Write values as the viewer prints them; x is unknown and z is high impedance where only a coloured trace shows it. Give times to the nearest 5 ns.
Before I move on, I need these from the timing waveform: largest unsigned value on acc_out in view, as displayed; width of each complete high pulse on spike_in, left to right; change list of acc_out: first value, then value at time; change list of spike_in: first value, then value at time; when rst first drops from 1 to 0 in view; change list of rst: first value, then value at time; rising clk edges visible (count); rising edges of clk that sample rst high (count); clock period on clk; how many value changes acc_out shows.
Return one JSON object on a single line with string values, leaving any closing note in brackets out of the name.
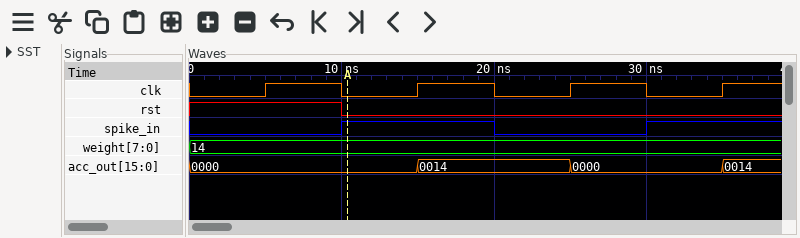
{"largest unsigned value on acc_out in view, as displayed": "0014", "width of each complete high pulse on spike_in, left to right": "10 ns", "change list of acc_out: first value, then value at time": "0000, 0014 at 15 ns, 0000 at 25 ns, 0014 at 35 ns", "change list of spike_in: first value, then value at time": "0, 1 at 10 ns, 0 at 20 ns, 1 at 30 ns", "when rst first drops from 1 to 0 in view": "10 ns", "change list of rst: first value, then value at time": "1, 0 at 10 ns", "rising clk edges visible": "4", "rising edges of clk that sample rst high": "1", "clock period on clk": "10 ns", "how many value changes acc_out shows": "3"}
